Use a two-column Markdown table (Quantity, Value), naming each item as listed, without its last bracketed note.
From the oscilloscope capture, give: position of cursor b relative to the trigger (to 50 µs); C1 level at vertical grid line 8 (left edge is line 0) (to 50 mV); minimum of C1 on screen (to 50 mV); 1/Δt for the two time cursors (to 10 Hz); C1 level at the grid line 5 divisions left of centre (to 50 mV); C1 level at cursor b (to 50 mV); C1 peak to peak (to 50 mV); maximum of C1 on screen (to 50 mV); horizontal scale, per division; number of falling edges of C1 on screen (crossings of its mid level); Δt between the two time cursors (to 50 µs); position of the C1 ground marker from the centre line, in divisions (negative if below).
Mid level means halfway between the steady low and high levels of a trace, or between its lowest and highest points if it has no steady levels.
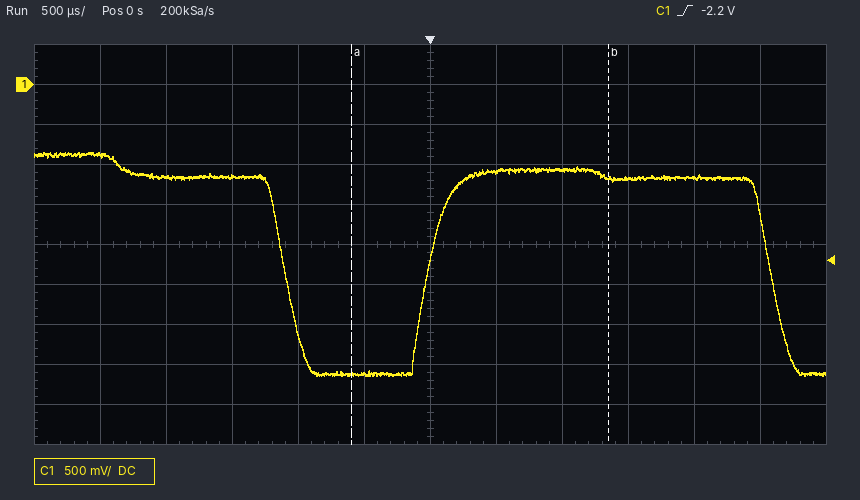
| Quantity | Value |
|---|---|
| position of cursor b relative to the trigger | +1.35 ms |
| C1 level at vertical grid line 8 (left edge is line 0) | -1.05 V |
| minimum of C1 on screen | -3.65 V |
| 1/Δt for the two time cursors | 510 Hz |
| C1 level at the grid line 5 divisions left of centre | -900 mV |
| C1 level at cursor b | -1.15 V |
| C1 peak to peak | 2.80 V |
| maximum of C1 on screen | -850 mV |
| horizontal scale, per division | 500 µs |
| number of falling edges of C1 on screen | 2 |
| Δt between the two time cursors | 1.95 ms |
| position of the C1 ground marker from the centre line, in divisions | +4.0 div |
